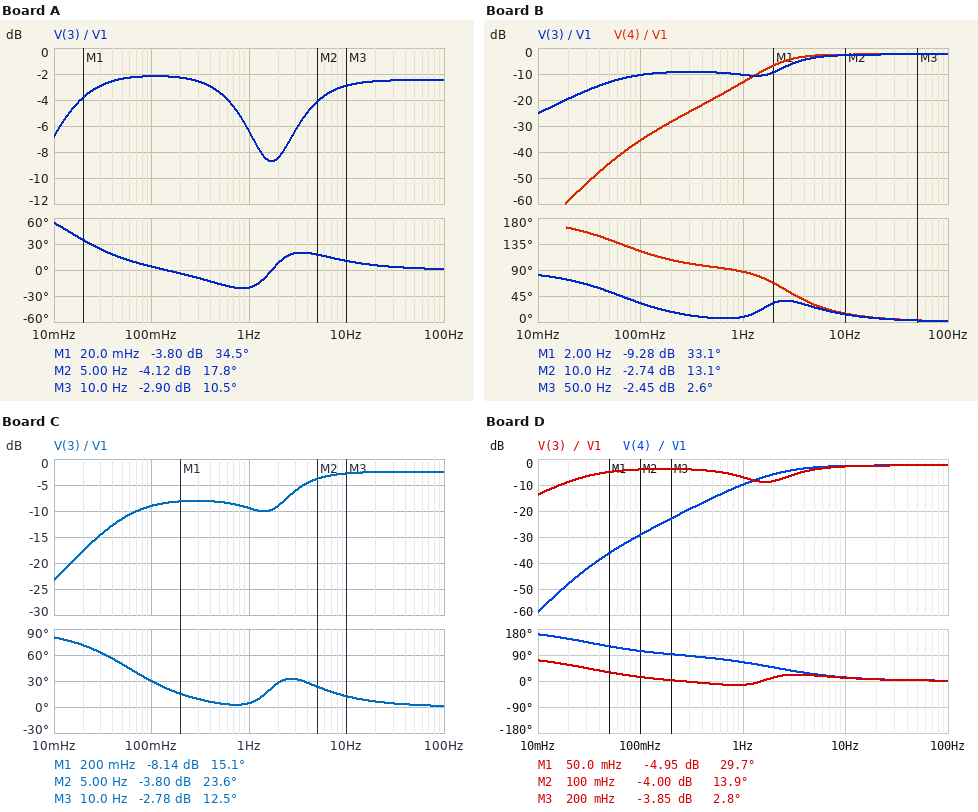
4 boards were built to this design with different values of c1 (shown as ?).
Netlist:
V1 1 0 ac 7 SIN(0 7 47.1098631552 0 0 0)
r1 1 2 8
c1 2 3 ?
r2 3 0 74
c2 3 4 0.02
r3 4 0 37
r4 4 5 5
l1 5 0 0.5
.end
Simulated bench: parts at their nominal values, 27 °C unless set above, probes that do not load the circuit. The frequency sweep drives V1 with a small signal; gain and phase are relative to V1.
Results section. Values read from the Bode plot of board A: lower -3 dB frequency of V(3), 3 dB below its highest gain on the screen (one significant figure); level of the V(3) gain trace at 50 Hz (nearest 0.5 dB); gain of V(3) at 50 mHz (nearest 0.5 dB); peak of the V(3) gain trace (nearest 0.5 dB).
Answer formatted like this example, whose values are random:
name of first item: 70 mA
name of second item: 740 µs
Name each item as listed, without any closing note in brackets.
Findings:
lower -3 dB frequency of V(3), 3 dB below its highest gain on the screen: 10 mHz
level of the V(3) gain trace at 50 Hz: -2.5 dB
gain of V(3) at 50 mHz: -2.5 dB
peak of the V(3) gain trace: -2.0 dB
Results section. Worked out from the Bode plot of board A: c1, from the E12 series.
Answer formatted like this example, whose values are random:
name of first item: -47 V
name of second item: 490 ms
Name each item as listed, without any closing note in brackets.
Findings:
c1, from the E12 series: 120 mF
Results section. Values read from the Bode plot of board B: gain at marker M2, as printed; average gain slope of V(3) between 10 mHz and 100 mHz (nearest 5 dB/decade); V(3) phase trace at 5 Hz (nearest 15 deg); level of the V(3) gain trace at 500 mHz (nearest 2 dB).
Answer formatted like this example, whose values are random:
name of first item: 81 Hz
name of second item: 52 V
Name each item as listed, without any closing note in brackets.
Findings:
gain at marker M2, as printed: -2.74 dB
average gain slope of V(3) between 10 mHz and 100 mHz: 15 dB/decade
V(3) phase trace at 5 Hz: 30 deg
level of the V(3) gain trace at 500 mHz: -10 dB
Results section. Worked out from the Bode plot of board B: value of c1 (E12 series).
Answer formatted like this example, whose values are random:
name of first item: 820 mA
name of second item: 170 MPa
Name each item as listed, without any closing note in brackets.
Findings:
value of c1: 12 mF
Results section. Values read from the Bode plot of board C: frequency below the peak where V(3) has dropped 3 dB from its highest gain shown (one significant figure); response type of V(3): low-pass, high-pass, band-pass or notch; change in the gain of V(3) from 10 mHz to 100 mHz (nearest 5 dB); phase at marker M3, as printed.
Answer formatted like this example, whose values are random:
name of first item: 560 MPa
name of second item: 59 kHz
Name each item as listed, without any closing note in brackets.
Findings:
frequency below the peak where V(3) has dropped 3 dB from its highest gain shown: 3 Hz
response type of V(3): low-pass, high-pass, band-pass or notch: high-pass
change in the gain of V(3) from 10 mHz to 100 mHz: 15 dB
phase at marker M3, as printed: 12.5 deg
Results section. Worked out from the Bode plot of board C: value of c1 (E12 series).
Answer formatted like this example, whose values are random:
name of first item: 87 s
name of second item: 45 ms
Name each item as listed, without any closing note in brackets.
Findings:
value of c1: 15 mF
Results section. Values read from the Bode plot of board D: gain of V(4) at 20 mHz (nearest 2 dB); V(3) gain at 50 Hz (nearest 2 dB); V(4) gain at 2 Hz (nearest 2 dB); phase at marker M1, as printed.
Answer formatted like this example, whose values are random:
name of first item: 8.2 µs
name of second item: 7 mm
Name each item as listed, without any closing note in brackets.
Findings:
gain of V(4) at 20 mHz: -48 dB
V(3) gain at 50 Hz: -2 dB
V(4) gain at 2 Hz: -6 dB
phase at marker M1, as printed: 29.7 deg
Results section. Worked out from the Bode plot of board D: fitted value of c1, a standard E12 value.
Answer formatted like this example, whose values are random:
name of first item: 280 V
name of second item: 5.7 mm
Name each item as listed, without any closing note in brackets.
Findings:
fitted value of c1, a standard E12 value: 47 mF
